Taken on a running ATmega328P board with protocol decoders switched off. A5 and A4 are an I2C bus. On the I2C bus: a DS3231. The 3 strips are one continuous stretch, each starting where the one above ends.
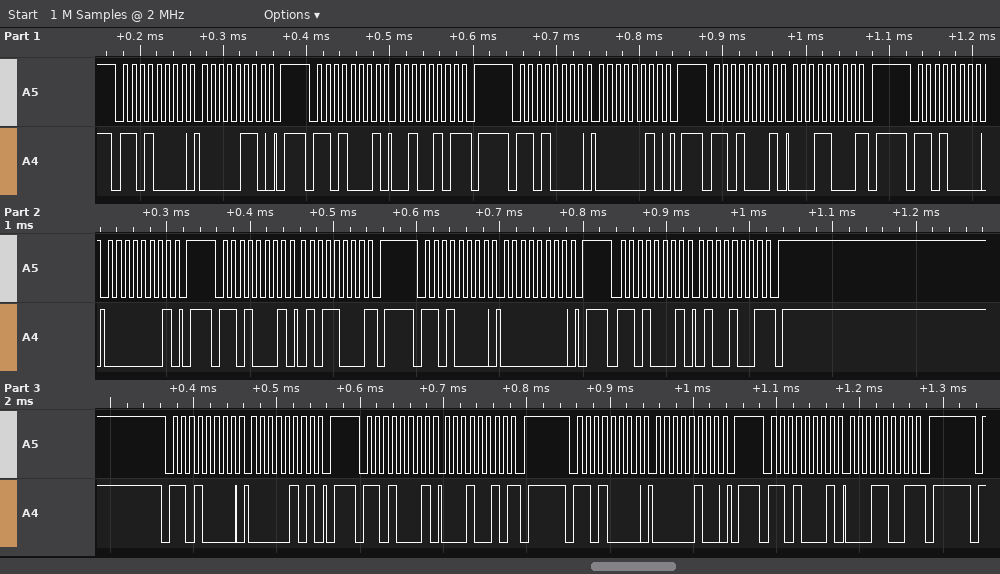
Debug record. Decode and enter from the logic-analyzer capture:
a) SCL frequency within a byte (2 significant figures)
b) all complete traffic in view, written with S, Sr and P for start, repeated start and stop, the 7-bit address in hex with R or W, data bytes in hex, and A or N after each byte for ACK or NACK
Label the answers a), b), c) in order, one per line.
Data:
a) 100 kHz
b) S 68W A 06 A P S 68R A 25 N P S 68W A 02 A P S 68R A 18 N P S 68W A 01 A P S 68R A 58 N P S 68W A 00 A P S 68R A 49 N P S 68W A 05 A P S 68R A 12 N P S 68W A 04 A P S 68R A 19 N P
